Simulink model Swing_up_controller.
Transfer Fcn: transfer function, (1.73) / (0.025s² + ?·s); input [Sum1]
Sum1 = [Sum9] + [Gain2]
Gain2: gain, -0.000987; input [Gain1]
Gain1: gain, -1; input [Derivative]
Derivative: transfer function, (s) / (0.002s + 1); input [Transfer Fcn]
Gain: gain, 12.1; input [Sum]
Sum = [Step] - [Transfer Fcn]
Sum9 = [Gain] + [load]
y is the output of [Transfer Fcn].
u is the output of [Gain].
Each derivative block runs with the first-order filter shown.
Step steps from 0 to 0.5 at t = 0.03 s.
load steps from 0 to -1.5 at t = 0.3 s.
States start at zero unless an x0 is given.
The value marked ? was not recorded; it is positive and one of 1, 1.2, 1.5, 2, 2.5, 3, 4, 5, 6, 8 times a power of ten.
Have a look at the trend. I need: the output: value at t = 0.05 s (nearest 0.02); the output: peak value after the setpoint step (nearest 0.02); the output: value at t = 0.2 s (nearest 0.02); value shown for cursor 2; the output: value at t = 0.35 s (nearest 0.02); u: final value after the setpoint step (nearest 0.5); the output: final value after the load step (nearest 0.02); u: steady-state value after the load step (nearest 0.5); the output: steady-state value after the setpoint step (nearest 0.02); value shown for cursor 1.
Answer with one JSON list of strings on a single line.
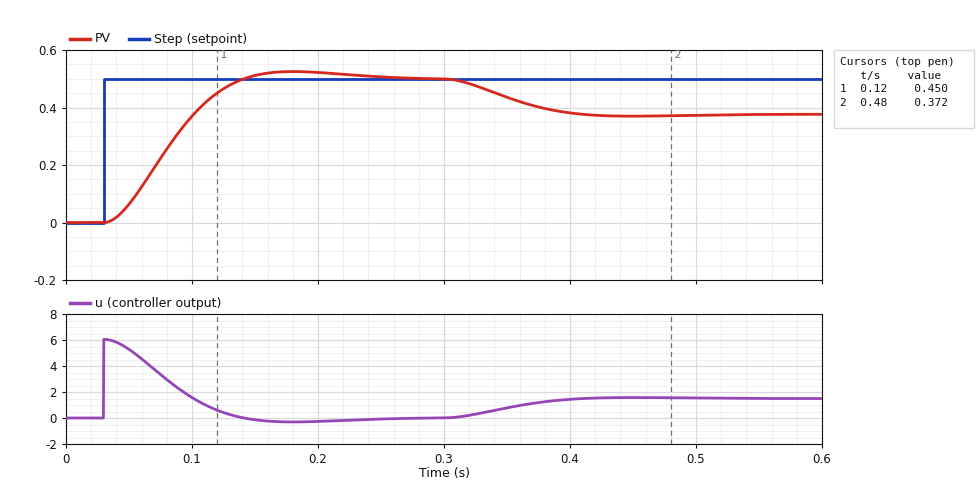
["0.06", "0.52", "0.52", "0.372", "0.44", "0.0", "0.38", "1.5", "0.50", "0.450"]
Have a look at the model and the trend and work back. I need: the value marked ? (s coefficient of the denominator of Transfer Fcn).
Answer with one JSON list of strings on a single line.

["1"]
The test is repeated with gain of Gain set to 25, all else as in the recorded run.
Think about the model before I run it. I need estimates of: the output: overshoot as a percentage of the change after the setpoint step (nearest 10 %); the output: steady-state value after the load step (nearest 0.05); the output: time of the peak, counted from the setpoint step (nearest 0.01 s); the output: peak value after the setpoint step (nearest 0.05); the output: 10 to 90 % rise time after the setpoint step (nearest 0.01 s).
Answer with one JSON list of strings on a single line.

["20 %", "0.45", "0.09 s", "0.60", "0.04 s"]
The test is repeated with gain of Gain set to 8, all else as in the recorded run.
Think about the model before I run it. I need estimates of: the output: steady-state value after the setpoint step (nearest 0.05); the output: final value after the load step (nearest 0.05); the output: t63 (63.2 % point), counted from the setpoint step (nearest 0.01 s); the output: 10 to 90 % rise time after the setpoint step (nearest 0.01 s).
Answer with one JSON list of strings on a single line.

["0.50", "0.30", "0.08 s", "0.11 s"]
